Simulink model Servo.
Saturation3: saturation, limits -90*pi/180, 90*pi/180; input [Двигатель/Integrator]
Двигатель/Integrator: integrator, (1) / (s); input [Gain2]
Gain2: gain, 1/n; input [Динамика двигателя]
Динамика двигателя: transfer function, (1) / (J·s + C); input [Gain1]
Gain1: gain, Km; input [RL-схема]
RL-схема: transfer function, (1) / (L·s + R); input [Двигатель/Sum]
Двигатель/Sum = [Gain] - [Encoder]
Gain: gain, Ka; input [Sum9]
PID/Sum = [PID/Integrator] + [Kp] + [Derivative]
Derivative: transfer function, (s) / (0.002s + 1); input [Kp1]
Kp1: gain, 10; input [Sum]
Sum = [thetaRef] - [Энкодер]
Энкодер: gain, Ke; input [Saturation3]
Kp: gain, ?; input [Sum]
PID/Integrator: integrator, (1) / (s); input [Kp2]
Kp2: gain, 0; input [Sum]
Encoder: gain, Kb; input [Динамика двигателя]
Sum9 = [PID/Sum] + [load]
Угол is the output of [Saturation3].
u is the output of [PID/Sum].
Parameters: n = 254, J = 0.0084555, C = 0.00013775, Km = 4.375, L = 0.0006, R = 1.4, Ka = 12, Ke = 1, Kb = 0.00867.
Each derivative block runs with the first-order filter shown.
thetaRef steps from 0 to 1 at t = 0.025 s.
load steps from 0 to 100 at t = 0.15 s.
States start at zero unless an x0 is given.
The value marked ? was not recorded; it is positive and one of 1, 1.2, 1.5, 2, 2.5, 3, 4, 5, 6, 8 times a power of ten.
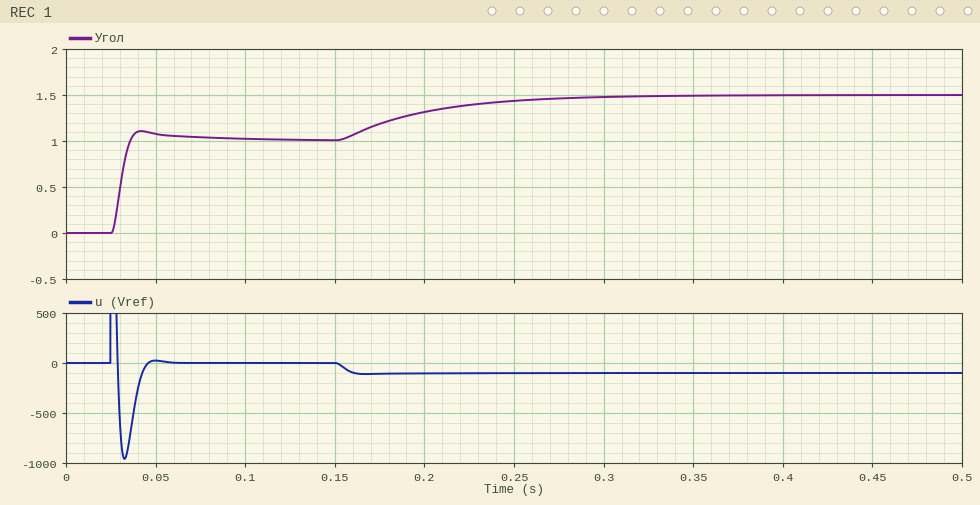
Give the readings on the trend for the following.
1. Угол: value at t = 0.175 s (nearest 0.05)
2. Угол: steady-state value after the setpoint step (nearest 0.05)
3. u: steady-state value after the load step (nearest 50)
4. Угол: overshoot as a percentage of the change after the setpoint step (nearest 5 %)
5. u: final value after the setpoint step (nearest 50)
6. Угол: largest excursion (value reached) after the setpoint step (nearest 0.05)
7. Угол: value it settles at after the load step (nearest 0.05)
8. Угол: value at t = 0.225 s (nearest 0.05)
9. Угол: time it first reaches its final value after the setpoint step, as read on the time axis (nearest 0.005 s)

1.20
1.00
-100
10 %
0
1.10
1.50
1.40
0.035 s
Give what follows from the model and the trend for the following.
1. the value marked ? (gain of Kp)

200
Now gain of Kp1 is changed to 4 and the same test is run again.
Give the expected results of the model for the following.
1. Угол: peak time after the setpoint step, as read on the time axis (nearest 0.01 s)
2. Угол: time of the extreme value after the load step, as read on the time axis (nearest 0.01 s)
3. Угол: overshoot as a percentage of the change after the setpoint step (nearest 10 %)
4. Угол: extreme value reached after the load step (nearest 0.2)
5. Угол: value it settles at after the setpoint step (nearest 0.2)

0.06 s
0.21 s
30 %
1.6
1.0
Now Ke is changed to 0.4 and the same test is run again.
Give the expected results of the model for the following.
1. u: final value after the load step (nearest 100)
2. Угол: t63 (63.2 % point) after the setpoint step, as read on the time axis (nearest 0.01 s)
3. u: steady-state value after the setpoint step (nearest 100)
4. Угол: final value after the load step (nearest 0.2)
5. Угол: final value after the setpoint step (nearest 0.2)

100
0.03 s
100
1.6
1.6
